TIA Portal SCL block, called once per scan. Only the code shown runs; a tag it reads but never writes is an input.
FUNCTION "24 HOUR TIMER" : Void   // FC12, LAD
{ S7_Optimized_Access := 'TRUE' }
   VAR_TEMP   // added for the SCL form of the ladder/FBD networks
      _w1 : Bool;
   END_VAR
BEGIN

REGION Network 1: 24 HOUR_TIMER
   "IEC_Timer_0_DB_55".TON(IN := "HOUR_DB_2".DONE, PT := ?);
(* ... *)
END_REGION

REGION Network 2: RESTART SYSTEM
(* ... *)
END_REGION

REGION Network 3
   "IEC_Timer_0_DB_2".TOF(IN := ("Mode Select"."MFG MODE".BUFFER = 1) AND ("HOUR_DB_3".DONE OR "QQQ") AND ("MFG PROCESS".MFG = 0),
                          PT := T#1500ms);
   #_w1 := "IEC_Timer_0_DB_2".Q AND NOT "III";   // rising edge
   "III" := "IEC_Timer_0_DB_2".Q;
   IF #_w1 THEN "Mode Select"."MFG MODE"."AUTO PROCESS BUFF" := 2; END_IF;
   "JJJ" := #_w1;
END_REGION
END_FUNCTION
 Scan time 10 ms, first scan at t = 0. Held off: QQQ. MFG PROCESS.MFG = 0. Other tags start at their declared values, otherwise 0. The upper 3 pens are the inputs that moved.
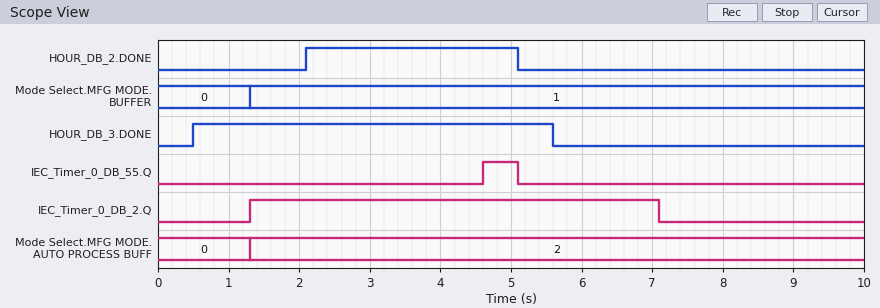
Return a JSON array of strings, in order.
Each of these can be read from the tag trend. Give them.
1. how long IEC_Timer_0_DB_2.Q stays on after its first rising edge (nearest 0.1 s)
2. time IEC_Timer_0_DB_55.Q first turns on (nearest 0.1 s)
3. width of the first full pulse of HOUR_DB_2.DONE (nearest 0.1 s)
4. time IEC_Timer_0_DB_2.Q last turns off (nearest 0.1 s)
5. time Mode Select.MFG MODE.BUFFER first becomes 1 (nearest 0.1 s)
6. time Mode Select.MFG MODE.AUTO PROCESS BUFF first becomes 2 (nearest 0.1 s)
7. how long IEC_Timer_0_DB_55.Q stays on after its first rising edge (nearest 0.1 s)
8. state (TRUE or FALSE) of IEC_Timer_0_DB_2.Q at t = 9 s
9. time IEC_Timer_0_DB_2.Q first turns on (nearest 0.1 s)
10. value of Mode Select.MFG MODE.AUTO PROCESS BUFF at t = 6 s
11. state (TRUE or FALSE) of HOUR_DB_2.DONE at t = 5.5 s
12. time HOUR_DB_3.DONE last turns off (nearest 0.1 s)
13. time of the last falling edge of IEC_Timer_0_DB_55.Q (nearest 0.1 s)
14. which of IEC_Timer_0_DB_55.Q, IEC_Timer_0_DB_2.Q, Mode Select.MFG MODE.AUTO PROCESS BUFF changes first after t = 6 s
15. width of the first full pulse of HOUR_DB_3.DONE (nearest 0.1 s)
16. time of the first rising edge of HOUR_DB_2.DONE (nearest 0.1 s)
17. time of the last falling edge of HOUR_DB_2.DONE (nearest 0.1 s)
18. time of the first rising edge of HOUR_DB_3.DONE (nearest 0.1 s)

["5.8 s", "4.6 s", "3.0 s", "7.1 s", "1.3 s", "1.3 s", "0.5 s", "FALSE", "1.3 s", "2", "FALSE", "5.6 s", "5.1 s", "IEC_Timer_0_DB_2.Q", "5.1 s", "2.1 s", "5.1 s", "0.5 s"]
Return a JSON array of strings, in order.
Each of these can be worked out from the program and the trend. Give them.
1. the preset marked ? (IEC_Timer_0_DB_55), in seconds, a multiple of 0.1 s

["2.5 s"]
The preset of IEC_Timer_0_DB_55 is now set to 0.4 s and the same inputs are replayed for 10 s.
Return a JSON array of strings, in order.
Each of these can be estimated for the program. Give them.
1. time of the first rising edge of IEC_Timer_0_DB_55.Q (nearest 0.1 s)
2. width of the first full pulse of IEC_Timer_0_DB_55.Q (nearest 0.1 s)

["2.5 s", "2.6 s"]
